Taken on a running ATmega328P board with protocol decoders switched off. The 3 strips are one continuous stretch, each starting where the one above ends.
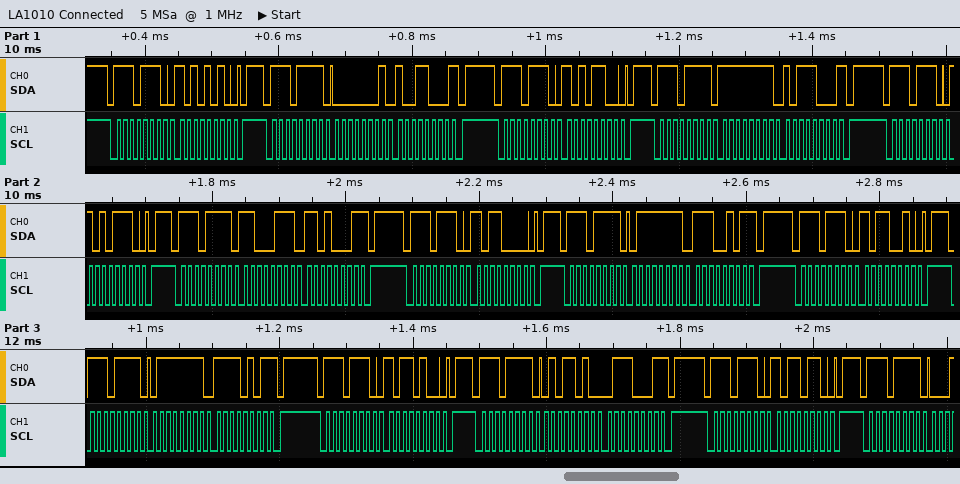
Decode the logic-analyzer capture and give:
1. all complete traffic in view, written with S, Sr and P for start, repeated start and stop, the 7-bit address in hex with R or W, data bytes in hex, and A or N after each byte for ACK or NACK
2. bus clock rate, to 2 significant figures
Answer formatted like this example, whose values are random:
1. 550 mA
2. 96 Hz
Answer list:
1. S 77W A AA A P S 77R A 01 A 98 N P S 77W A AC A P S 77R A FF A B8 N P S 77W A AE A P S 77R A C7 A D1 N P S 77W A B0 A P S 77R A 7F A E5 N P S 77W A B2 A P S 77R A 7F A F5 N P S 77W A B4 A P S 77R A 5A A 71 N P S 77W A B6 A P S 77R A
2. 100 kHz
